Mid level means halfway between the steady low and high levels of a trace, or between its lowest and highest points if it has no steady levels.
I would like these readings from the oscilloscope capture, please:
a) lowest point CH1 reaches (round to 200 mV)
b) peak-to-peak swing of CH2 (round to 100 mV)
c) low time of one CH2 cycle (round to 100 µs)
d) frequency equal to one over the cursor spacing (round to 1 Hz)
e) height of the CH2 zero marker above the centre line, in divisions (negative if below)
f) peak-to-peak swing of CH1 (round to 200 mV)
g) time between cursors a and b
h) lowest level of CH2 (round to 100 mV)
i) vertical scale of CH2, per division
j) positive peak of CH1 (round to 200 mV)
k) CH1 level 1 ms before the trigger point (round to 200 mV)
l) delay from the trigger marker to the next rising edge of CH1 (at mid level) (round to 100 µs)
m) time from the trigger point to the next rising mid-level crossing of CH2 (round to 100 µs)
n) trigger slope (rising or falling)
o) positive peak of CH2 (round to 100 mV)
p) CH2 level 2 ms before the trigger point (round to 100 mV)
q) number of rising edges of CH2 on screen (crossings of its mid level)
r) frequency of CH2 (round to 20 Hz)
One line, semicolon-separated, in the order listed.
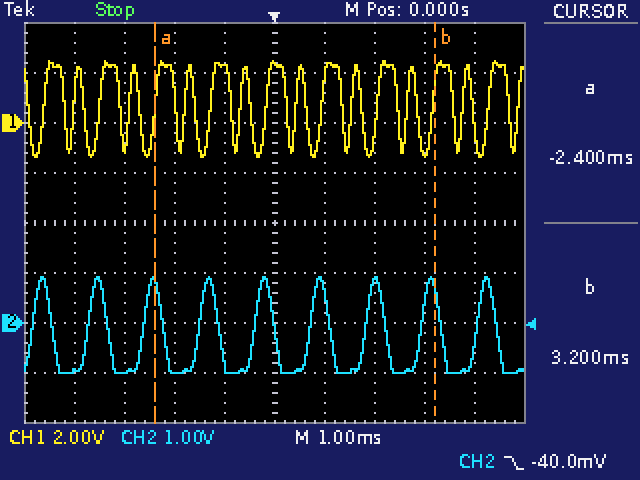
-1.4 V; 1.9 V; 700 µs; 179 Hz; -2.0 div; 3.8 V; 5.6 ms; -1.0 V; 1 V; 2.4 V; 2.2 V; 400 µs; 700 µs; falling; 900 mV; -1.0 V; 9; 900 Hz
